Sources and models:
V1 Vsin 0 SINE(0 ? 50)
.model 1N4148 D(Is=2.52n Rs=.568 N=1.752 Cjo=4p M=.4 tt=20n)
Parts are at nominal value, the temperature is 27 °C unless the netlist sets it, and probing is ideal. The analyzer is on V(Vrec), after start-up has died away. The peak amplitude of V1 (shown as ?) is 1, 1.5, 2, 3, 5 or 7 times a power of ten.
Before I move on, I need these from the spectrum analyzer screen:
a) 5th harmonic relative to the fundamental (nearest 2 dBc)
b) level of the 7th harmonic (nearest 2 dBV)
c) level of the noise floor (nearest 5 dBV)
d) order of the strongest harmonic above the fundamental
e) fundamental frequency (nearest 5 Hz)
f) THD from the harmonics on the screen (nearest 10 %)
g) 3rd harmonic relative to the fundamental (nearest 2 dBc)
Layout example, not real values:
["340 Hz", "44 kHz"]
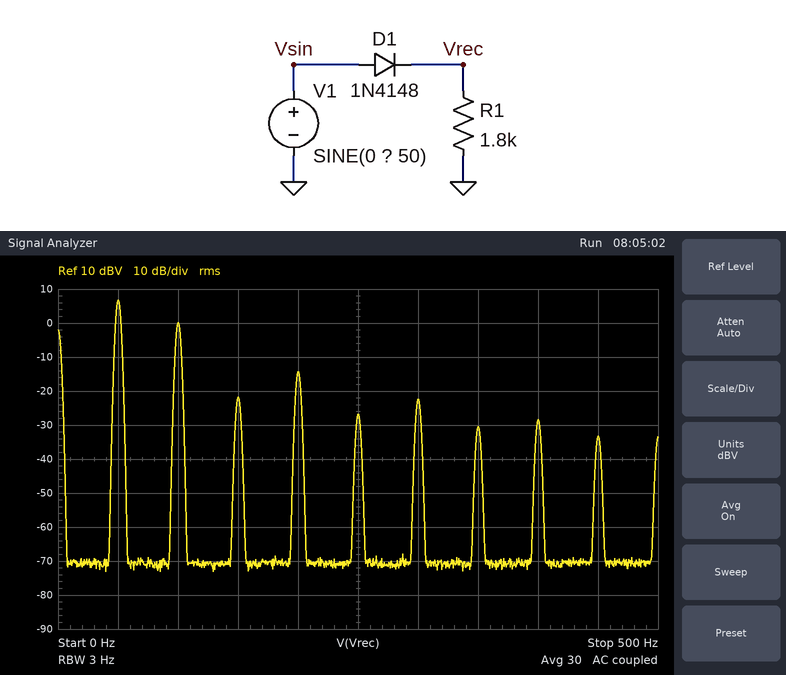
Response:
["-34 dBc", "-30 dBV", "-70 dBV", "2", "50 Hz", "50 %", "-28 dBc"]
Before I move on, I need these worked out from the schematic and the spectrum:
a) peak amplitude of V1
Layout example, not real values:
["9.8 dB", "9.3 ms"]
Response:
["7 V"]
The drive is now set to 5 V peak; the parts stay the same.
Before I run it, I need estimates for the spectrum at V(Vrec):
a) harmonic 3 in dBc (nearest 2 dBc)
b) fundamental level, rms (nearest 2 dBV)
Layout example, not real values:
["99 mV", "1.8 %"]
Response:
["-26 dBc", "4 dBV"]
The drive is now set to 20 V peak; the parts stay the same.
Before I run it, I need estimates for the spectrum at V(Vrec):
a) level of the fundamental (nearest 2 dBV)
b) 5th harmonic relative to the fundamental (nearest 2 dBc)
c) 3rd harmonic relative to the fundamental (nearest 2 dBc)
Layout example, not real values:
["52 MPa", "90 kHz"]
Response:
["16 dBV", "-42 dBc", "-38 dBc"]
